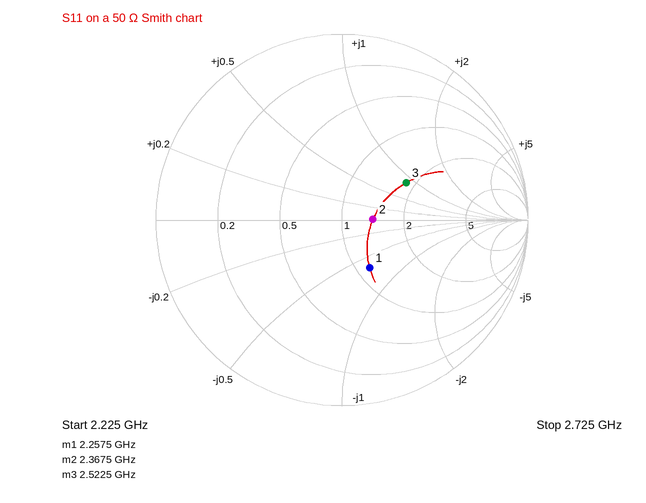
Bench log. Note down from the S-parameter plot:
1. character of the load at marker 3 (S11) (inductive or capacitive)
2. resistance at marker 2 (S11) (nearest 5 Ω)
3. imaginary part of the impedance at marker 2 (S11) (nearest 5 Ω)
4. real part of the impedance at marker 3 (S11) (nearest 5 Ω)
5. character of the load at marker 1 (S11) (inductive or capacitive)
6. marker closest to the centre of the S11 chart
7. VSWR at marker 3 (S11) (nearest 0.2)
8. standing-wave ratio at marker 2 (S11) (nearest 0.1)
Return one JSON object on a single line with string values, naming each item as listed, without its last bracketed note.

{"character of the load at marker 3 (S11)": "inductive", "resistance at marker 2 (S11)": "70 Ω", "imaginary part of the impedance at marker 2 (S11)": "0 Ω", "real part of the impedance at marker 3 (S11)": "90 Ω", "character of the load at marker 1 (S11)": "capacitive", "marker closest to the centre of the S11 chart": "marker 2", "VSWR at marker 3 (S11)": "2.4", "standing-wave ratio at marker 2 (S11)": "1.4"}
